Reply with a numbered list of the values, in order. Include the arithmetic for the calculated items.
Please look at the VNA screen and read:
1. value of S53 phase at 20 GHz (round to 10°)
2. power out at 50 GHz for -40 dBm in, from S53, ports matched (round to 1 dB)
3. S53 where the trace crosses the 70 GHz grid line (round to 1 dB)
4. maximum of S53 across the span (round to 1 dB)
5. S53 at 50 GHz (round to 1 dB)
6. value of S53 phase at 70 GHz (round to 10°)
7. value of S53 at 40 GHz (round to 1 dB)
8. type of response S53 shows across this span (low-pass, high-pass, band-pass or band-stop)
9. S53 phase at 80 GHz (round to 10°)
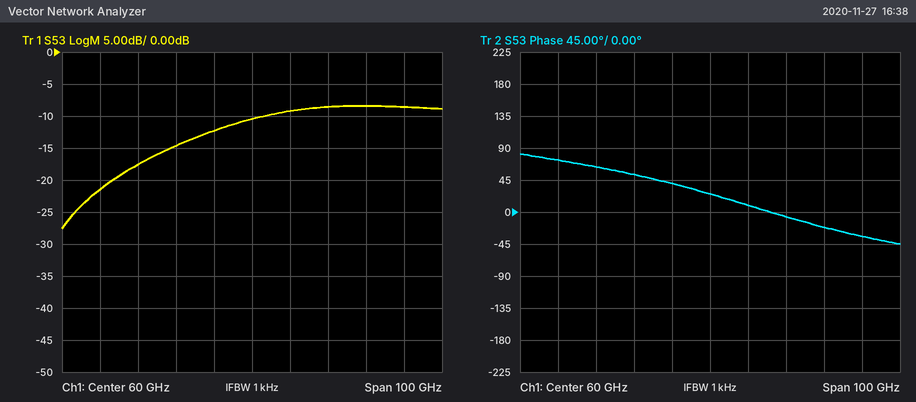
1. 70°
2. -40 dBm + (-12 dB) = -52 dBm
3. -9 dB
4. -8 dB
5. -12 dB
6. 10°
7. -15 dB
8. high-pass
9. -10°
